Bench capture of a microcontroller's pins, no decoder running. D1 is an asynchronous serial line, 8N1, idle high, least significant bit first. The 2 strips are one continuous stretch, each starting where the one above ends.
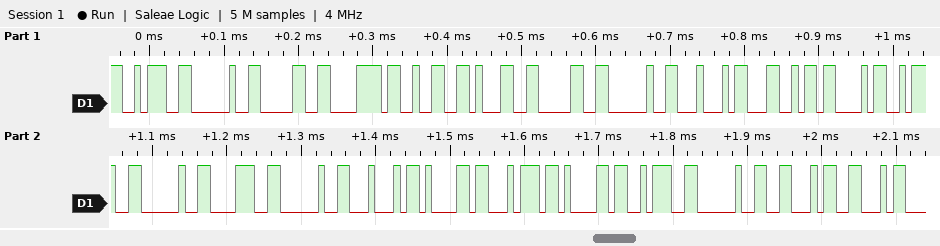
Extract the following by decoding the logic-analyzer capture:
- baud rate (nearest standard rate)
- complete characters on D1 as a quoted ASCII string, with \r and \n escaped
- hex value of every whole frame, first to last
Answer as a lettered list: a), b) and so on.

a) 115200 baud
b) ": 0x210 DLC: 8 Data: FF"
c) 3A 20 30 78 32 31 30 20 44 4C 43 3A 20 38 20 44 61 74 61 3A 20 46 46
